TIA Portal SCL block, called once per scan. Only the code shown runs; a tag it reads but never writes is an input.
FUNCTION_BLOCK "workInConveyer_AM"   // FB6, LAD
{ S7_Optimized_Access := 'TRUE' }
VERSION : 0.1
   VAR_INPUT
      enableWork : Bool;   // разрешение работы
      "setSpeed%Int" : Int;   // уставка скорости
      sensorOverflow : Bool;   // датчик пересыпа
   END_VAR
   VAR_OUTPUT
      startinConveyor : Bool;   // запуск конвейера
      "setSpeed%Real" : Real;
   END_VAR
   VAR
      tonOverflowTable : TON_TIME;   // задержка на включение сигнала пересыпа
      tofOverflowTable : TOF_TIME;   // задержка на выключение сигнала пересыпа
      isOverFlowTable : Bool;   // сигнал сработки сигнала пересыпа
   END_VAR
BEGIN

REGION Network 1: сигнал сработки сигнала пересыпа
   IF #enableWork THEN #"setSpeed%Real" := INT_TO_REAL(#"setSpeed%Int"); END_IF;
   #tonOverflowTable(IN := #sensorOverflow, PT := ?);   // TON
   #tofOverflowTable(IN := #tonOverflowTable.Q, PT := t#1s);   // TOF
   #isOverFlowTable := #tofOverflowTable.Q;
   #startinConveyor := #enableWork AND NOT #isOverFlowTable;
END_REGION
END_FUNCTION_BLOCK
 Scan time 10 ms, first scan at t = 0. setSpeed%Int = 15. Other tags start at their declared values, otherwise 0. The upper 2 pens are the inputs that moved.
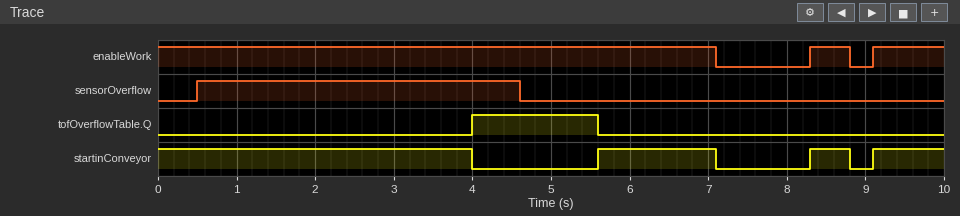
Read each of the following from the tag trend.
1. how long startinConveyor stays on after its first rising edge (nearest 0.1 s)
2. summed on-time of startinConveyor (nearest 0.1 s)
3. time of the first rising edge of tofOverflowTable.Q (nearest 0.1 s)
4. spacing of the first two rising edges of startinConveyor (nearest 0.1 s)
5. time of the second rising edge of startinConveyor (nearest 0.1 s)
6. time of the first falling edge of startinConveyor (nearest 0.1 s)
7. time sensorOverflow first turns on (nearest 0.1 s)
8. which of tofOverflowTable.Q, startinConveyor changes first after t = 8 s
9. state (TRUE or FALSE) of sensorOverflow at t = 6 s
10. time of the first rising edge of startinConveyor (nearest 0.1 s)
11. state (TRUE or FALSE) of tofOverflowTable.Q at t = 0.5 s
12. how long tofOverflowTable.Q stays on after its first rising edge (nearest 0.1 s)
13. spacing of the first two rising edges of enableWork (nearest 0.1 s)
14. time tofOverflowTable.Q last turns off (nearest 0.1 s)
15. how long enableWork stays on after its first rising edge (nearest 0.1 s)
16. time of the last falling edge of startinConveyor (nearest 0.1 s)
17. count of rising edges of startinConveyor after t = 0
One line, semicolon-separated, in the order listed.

1.5 s; 6.9 s; 4.0 s; 2.7 s; 8.3 s; 4.0 s; 0.5 s; startinConveyor; FALSE; 5.6 s; FALSE; 1.6 s; 0.8 s; 5.6 s; 0.5 s; 8.8 s; 3
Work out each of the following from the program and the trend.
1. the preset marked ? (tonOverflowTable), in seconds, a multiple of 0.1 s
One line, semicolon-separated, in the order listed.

3.5 s
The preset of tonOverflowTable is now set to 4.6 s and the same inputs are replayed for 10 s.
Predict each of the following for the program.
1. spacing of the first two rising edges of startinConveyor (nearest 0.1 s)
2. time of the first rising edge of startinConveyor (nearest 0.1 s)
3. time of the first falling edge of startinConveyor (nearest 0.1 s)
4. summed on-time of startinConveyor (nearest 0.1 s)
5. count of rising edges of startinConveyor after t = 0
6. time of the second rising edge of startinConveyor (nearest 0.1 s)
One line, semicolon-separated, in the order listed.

0.8 s; 8.3 s; 7.1 s; 8.5 s; 2; 9.1 s
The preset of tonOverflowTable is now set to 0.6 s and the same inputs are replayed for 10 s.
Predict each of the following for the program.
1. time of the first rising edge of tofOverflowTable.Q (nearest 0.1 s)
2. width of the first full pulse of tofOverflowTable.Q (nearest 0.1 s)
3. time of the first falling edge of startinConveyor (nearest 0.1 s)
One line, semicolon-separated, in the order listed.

1.1 s; 4.5 s; 1.1 s
